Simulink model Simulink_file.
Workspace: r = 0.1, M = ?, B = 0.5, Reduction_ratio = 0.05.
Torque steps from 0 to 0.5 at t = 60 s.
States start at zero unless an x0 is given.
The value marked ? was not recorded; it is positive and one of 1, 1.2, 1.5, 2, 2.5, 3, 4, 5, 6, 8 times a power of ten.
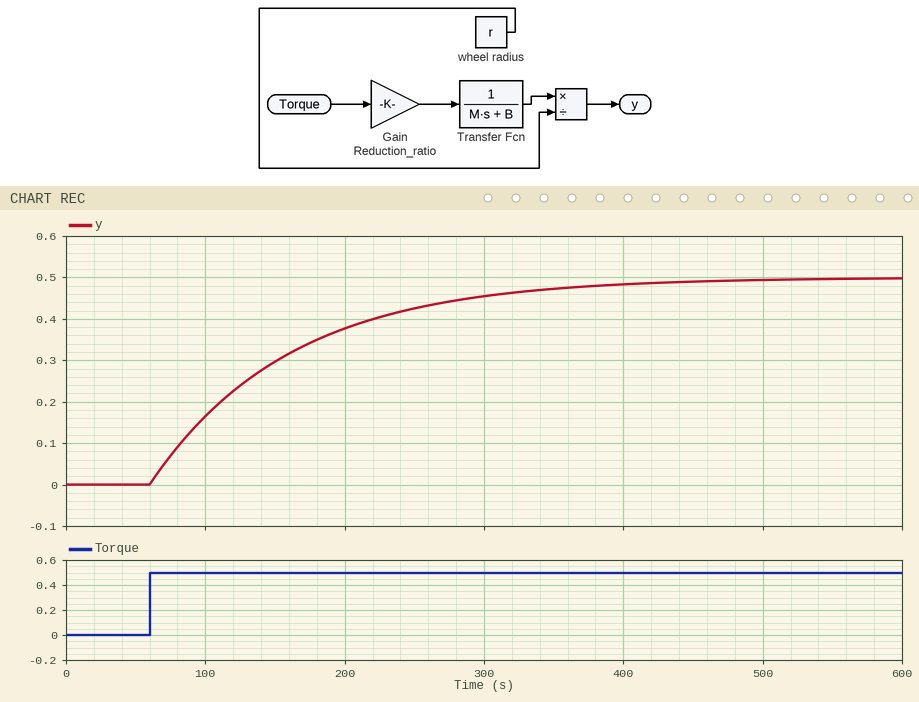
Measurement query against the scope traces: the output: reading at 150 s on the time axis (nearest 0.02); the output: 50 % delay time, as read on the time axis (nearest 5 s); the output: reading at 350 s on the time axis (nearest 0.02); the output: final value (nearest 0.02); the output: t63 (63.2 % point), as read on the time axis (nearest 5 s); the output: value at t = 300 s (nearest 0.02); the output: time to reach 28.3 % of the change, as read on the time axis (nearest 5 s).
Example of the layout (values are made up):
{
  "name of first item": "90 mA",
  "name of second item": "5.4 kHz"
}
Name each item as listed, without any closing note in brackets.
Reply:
{
  "the output: reading at 150 s on the time axis": "0.30",
  "the output: 50 % delay time, as read on the time axis": "130 s",
  "the output: reading at 350 s on the time axis": "0.48",
  "the output: final value": "0.50",
  "the output: t63 (63.2 % point), as read on the time axis": "160 s",
  "the output: value at t = 300 s": "0.46",
  "the output: time to reach 28.3 % of the change, as read on the time axis": "95 s"
}
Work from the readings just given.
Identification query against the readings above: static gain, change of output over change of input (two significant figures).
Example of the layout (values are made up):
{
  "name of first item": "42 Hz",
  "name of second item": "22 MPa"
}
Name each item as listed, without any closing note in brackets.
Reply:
{
  "static gain, change of output over change of input": "1.0"
}
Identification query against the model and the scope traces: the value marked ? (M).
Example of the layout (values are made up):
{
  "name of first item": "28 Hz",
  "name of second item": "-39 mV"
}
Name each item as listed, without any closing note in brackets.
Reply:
{
  "the value marked ?": "50"
}
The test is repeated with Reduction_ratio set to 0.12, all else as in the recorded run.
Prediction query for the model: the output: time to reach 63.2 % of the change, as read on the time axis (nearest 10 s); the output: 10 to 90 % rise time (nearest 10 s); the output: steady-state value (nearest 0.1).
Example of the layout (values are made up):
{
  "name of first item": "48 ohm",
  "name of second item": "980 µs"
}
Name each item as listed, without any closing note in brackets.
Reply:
{
  "the output: time to reach 63.2 % of the change, as read on the time axis": "160 s",
  "the output: 10 to 90 % rise time": "220 s",
  "the output: steady-state value": "1.2"
}
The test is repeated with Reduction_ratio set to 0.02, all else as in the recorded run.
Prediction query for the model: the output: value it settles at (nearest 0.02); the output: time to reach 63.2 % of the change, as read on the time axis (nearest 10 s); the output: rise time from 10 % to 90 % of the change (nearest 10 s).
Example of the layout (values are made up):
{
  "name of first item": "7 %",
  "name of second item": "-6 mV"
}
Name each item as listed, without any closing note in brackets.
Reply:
{
  "the output: value it settles at": "0.20",
  "the output: time to reach 63.2 % of the change, as read on the time axis": "160 s",
  "the output: rise time from 10 % to 90 % of the change": "220 s"
}
